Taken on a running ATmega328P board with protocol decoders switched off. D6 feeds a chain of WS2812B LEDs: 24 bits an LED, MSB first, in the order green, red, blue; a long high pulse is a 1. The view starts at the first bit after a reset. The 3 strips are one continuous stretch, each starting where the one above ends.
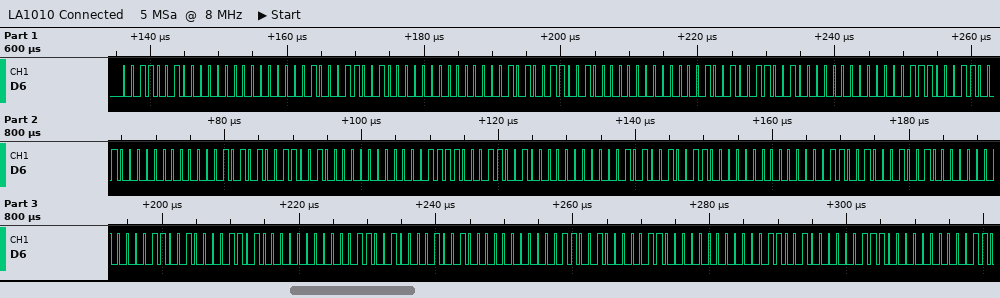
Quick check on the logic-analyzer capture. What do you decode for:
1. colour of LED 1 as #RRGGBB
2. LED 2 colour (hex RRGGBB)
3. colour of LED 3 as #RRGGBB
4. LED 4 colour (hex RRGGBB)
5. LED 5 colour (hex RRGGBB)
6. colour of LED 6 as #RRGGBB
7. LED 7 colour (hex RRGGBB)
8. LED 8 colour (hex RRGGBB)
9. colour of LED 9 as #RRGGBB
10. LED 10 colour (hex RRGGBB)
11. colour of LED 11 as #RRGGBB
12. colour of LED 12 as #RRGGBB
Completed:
#003202
#003205
#003209
#00320E
#003215
#00321E
#003229
#003032
#002432
#001A32
#001232
#000C32
